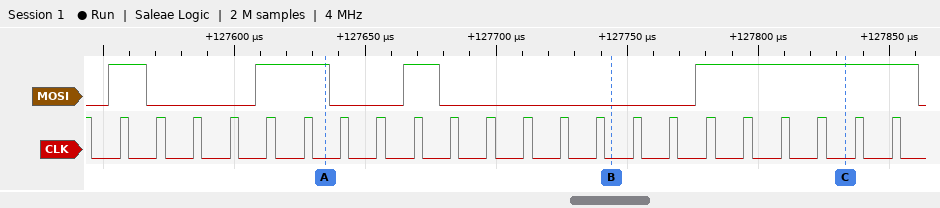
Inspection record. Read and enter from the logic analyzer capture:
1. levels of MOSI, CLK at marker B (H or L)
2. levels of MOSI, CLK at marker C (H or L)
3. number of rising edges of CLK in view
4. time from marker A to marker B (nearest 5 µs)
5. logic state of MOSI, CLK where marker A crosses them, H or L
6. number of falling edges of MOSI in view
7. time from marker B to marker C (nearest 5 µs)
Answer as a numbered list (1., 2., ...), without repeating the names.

1. MOSI=L, CLK=L
2. MOSI=H, CLK=L
3. 22
4. 110 µs
5. MOSI=H, CLK=L
6. 4
7. 90 µs
